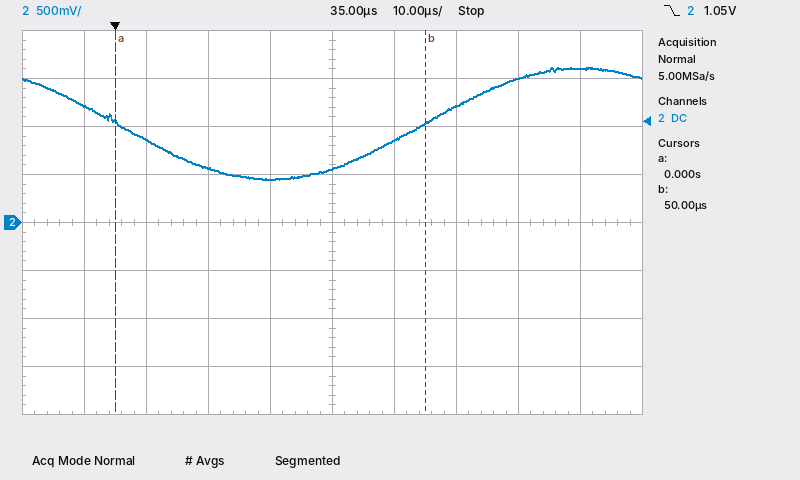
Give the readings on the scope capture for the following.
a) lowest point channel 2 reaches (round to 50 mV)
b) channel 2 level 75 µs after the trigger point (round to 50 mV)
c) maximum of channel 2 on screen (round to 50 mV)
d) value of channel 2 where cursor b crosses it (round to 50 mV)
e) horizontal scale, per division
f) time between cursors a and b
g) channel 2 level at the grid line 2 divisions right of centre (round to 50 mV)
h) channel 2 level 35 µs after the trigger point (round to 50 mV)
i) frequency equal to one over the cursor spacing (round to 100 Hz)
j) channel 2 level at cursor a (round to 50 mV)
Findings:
450 mV
1.60 V
1.60 V
1.05 V
10 µs
50 µs
1.20 V
550 mV
20.0 kHz
1.05 V
